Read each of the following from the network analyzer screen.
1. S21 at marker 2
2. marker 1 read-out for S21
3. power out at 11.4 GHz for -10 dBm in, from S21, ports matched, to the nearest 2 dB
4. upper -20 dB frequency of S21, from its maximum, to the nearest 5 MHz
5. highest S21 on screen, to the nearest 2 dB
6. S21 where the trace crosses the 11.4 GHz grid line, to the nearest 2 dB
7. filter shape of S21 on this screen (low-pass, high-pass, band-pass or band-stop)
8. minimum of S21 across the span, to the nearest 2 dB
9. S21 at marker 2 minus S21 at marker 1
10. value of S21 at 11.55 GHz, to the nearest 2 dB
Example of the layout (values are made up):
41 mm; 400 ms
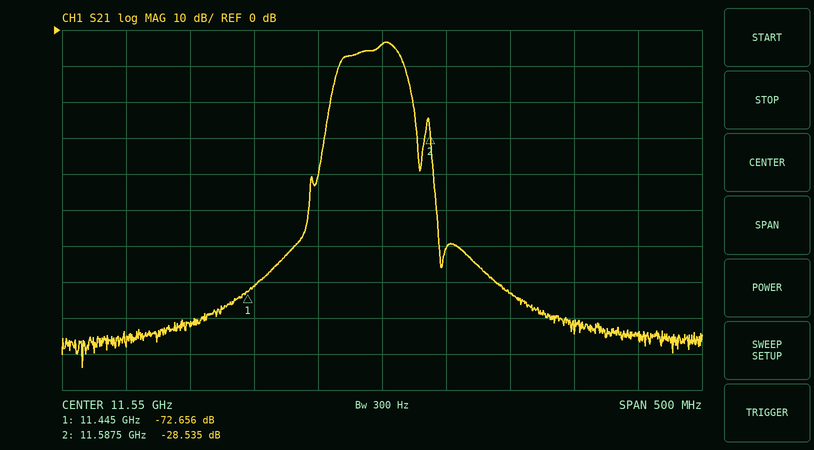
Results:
-28.535 dB; -72.656 dB; -92 dBm; 11.575 GHz; -4 dB; -82 dB; band-pass; -94 dB; 44.121 dB; -4 dB
